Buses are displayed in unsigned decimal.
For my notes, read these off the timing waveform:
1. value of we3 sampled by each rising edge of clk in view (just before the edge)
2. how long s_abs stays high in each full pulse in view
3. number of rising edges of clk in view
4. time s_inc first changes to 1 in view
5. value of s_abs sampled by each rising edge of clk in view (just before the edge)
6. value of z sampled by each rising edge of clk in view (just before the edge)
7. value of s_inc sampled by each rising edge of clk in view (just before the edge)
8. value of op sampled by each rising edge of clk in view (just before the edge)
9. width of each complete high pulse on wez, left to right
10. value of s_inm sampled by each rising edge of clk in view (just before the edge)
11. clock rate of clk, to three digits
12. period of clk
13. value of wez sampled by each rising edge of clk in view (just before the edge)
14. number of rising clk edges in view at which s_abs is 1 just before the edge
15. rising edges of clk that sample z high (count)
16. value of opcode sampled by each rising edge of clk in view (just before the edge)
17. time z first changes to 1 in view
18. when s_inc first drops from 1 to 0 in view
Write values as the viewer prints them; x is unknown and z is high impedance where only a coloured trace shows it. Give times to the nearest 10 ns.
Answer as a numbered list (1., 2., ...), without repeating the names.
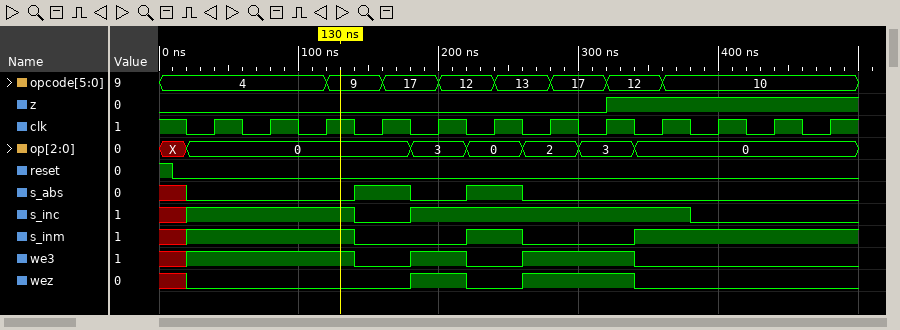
1. 1 1 1 0 1 0 1 1 0 0 0 0
2. 40 ns, 40 ns
3. 12
4. 20 ns
5. 0 0 0 1 0 1 0 0 0 0 0 0
6. 0 0 0 0 0 0 0 0 1 1 1 1
7. 1 1 1 0 1 1 1 1 1 0 0 0
8. 0, 0, 0, 0, 3, 0, 2, 3, 0, 0, 0, 0
9. 40 ns, 80 ns
10. 1 1 1 0 0 1 0 0 1 1 1 1
11. 25.0 MHz
12. 40 ns
13. 0 0 0 0 1 0 1 1 0 0 0 0
14. 2
15. 4
16. 4, 4, 4, 9, 17, 12, 13, 17, 12, 10, 10, 10
17. 320 ns
18. 140 ns
